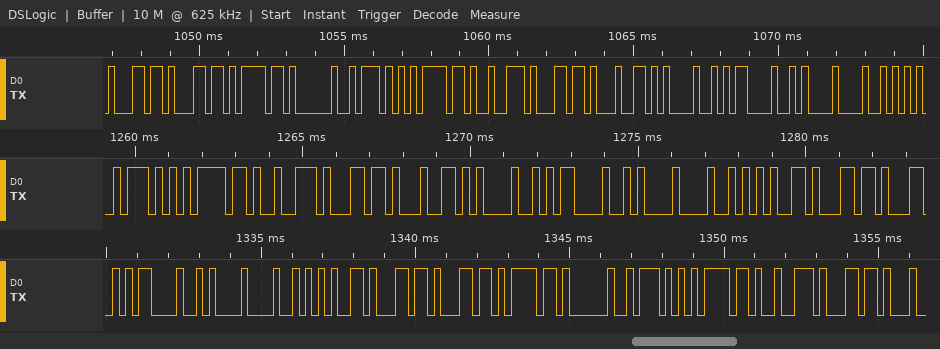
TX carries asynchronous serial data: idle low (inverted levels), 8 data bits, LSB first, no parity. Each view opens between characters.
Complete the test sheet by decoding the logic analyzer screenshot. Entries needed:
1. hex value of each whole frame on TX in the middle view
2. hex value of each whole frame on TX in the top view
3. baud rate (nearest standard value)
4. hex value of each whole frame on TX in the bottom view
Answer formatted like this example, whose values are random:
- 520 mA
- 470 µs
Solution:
- 51, 21, 1B, 27, 37, BD, E5, EB, 6F, 35, 27
- 27, 27, 21, BF, 51, 21, 1B, 27, 37, BD, E5, EB, 6F
- 4800 baud
- E5, EB, 6F, 35, 27, 27, 21, BF, 51, 21, 1B, 27
